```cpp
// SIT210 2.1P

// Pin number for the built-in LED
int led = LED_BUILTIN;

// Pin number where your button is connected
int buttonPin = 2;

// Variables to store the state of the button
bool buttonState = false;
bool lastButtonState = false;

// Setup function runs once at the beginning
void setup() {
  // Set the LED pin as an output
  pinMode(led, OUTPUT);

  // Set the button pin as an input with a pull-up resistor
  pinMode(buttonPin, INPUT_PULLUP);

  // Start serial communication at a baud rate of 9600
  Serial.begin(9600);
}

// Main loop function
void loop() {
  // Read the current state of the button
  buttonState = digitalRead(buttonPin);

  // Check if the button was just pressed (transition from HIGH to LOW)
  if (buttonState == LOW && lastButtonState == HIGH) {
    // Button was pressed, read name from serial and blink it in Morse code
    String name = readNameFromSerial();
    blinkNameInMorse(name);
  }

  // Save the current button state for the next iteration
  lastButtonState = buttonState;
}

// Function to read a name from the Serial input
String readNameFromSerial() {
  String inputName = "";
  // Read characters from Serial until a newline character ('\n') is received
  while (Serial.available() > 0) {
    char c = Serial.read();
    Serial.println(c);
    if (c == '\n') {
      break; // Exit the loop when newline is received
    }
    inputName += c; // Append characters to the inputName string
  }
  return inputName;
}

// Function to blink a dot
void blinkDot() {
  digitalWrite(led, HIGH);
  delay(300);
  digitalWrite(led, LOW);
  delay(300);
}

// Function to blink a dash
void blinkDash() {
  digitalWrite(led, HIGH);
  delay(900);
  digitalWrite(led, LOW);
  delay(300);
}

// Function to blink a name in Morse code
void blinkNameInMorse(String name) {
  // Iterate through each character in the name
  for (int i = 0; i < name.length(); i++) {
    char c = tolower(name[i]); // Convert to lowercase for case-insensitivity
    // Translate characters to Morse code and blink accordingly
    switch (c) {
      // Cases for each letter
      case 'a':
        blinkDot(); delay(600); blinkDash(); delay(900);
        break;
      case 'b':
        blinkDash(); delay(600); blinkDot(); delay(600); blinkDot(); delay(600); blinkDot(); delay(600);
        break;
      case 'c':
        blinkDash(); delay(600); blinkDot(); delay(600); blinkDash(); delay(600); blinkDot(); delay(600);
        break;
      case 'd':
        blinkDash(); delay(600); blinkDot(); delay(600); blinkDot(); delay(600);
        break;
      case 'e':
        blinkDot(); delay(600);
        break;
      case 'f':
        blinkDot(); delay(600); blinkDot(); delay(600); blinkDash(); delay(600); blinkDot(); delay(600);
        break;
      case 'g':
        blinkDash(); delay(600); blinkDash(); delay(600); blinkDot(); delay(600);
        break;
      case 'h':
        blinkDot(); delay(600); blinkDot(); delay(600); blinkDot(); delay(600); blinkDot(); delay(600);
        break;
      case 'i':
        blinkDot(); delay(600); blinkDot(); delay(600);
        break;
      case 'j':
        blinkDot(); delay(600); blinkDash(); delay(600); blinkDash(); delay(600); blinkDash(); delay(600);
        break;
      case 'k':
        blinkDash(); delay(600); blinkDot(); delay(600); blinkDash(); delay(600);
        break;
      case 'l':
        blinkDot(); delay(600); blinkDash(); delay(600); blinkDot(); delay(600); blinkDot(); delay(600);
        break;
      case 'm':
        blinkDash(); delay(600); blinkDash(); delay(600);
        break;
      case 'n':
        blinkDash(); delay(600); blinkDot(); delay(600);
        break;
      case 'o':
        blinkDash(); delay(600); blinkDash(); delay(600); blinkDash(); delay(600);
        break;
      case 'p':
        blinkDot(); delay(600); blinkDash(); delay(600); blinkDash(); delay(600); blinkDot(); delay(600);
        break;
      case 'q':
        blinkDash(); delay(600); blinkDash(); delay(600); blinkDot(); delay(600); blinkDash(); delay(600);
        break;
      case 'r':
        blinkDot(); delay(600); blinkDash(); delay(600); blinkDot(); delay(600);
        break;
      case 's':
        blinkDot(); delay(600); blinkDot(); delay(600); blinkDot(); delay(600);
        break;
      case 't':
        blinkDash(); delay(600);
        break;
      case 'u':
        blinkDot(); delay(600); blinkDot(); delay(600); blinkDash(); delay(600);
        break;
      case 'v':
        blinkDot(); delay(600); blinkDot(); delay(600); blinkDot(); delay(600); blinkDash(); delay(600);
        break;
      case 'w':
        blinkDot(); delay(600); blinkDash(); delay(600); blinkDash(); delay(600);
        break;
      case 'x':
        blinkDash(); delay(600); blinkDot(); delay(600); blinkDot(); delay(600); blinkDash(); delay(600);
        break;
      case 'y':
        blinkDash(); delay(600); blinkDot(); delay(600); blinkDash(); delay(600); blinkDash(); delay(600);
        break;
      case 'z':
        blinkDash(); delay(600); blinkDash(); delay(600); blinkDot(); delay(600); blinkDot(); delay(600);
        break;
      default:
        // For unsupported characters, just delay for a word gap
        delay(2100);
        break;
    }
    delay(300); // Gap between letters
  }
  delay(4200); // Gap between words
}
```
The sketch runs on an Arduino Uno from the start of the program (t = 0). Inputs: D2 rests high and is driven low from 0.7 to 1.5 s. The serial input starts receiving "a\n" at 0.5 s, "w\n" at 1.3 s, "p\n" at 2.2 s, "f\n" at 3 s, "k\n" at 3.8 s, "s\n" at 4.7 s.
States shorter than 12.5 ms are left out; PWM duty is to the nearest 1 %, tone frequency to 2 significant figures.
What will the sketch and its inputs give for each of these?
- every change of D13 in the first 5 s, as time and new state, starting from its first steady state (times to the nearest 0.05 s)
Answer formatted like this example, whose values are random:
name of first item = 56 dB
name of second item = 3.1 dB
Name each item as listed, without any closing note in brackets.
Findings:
every change of D13 in the first 5 s, as time and new state, starting from its first steady state = 0 s low; 0.7 s high; 1 s low; 1.9 s high; 2.8 s low
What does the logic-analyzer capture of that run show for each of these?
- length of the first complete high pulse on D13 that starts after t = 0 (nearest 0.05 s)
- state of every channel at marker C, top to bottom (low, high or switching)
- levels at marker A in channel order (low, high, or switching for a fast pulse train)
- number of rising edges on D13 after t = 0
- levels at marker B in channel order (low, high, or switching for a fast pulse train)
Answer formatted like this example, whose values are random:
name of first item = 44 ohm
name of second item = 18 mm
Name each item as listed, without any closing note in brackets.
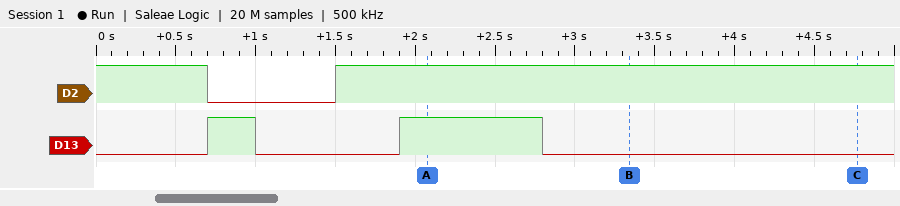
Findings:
length of the first complete high pulse on D13 that starts after t = 0 = 0.30 s
state of every channel at marker C, top to bottom = D2 high, D13 low
levels at marker A in channel order = D2 high, D13 high
number of rising edges on D13 after t = 0 = 2
levels at marker B in channel order = D2 high, D13 low
